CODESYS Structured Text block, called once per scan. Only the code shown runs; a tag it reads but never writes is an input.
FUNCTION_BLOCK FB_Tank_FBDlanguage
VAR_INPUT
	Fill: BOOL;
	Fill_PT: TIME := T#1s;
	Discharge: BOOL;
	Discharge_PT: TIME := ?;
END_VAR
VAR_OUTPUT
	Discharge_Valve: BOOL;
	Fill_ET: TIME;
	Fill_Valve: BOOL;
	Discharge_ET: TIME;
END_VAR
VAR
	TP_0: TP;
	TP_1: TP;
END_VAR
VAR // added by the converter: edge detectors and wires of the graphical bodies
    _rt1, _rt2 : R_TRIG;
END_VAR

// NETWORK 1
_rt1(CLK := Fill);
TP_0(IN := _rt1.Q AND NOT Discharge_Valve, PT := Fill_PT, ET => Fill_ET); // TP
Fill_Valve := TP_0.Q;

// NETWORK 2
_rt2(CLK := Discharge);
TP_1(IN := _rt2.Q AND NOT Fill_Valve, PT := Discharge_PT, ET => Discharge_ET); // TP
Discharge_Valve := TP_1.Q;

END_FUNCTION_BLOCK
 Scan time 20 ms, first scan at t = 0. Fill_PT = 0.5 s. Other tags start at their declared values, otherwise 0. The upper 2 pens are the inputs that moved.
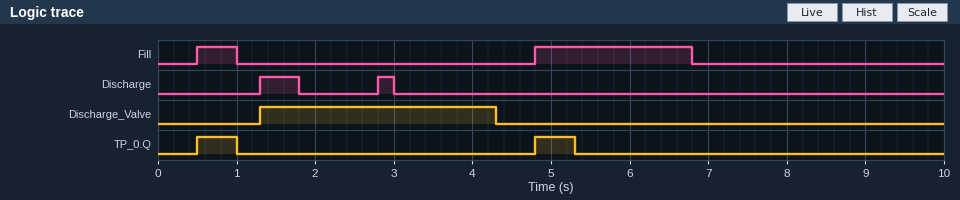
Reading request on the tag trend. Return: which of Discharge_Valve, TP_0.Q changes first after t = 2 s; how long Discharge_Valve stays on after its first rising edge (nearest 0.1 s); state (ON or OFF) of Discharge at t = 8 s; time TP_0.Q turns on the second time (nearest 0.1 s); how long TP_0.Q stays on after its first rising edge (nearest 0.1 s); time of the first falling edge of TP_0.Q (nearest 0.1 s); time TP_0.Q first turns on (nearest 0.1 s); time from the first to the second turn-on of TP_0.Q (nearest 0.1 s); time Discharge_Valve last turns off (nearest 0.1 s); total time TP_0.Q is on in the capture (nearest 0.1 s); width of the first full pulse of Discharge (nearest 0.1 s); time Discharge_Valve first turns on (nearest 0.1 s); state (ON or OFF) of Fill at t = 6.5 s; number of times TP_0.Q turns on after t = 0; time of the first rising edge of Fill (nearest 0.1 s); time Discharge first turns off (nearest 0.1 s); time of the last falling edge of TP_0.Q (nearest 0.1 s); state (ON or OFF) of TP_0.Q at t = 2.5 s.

Discharge_Valve
3.0 s
OFF
4.8 s
0.5 s
1.0 s
0.5 s
4.3 s
4.3 s
1.0 s
0.5 s
1.3 s
ON
2
0.5 s
1.8 s
5.3 s
OFF
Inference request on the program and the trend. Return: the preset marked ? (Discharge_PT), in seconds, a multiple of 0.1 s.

3.0 s
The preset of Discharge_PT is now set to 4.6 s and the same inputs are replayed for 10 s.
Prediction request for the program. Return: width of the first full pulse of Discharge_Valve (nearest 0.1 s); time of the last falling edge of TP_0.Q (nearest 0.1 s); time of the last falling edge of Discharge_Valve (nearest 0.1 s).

4.6 s
1.0 s
5.9 s
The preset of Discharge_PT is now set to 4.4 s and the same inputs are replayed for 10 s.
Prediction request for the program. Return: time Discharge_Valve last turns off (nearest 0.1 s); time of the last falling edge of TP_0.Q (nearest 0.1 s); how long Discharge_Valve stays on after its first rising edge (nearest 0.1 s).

5.7 s
1.0 s
4.4 s
